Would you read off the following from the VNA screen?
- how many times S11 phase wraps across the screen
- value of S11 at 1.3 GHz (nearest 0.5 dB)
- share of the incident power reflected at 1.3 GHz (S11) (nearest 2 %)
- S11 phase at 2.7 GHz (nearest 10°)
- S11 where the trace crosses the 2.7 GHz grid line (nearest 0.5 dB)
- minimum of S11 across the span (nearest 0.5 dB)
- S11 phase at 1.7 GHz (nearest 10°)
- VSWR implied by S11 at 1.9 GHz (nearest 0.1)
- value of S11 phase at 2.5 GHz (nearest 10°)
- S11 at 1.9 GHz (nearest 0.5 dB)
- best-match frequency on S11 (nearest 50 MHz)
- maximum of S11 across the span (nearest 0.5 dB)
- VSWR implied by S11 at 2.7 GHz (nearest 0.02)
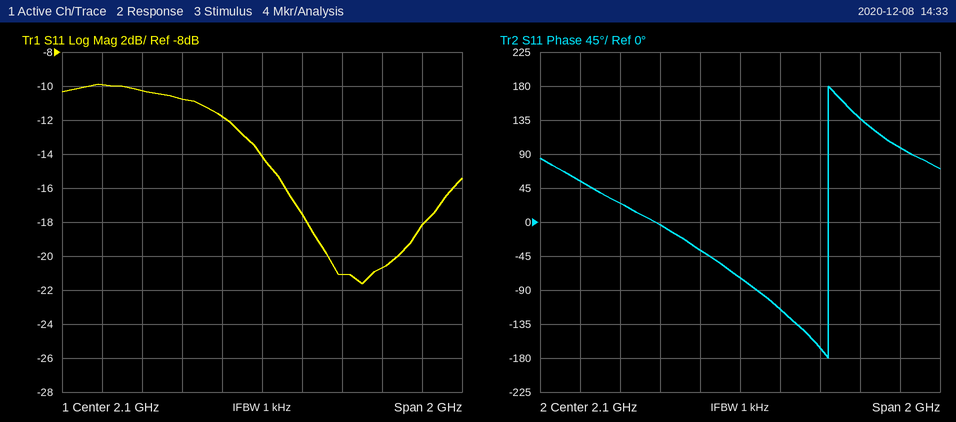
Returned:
1
-10.0 dB
10 %
140°
-20.5 dB
-21.5 dB
0°
1.7
-170°
-12.0 dB
2.60 GHz
-10.0 dB
1.20
